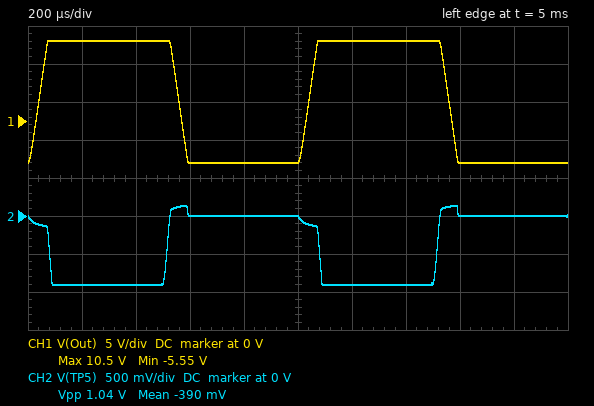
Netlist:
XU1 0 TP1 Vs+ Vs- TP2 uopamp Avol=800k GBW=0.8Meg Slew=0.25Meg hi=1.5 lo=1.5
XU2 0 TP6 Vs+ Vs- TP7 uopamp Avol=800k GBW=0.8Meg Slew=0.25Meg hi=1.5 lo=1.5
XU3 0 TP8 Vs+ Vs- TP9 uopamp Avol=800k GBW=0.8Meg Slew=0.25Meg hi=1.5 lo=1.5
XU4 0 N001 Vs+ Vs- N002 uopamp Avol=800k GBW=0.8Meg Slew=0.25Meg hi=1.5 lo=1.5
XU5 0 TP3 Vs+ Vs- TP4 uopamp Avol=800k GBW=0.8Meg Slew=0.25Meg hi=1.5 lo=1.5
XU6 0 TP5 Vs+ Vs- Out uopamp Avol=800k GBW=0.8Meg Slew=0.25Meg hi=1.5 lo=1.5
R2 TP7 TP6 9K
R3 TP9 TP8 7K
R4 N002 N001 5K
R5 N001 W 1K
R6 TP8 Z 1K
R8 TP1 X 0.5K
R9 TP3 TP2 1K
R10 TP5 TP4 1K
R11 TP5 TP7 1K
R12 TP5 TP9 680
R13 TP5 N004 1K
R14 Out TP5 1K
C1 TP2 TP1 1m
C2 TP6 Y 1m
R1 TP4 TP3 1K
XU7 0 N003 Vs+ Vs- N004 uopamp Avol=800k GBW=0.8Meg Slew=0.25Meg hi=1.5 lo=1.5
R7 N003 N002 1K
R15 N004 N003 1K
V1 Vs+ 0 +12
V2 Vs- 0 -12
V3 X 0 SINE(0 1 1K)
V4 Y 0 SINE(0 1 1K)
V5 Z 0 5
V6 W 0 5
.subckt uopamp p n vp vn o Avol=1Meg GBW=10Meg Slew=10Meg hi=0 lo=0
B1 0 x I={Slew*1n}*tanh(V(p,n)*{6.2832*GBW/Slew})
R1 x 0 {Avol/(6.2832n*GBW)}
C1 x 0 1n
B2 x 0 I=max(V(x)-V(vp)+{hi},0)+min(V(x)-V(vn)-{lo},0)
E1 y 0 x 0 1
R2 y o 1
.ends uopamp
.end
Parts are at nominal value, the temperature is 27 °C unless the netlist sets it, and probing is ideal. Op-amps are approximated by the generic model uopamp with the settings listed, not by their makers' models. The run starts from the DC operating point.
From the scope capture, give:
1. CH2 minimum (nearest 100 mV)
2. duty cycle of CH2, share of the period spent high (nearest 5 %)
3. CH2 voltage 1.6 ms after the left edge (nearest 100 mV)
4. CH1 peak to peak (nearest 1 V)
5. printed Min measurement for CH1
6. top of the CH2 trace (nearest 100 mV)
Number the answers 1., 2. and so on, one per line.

1. -900 mV
2. 55 %
3. 0 V
4. 16 V
5. -5.55 V
6. 100 mV
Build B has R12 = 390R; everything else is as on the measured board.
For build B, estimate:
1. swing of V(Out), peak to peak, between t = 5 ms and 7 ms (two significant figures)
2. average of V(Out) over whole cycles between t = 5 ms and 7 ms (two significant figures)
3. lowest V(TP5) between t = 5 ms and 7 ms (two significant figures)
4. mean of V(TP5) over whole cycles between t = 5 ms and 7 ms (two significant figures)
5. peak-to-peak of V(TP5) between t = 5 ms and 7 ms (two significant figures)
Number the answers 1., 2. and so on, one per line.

1. 4.6 V
2. 8.5 V
3. -2.5 V
4. -1.2 V
5. 2.6 V
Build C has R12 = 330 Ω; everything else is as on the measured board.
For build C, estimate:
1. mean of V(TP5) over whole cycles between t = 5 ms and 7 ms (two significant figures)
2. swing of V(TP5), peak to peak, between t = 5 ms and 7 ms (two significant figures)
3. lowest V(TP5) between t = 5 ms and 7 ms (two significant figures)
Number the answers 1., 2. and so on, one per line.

1. -1.5 V
2. 3.0 V
3. -3.0 V
